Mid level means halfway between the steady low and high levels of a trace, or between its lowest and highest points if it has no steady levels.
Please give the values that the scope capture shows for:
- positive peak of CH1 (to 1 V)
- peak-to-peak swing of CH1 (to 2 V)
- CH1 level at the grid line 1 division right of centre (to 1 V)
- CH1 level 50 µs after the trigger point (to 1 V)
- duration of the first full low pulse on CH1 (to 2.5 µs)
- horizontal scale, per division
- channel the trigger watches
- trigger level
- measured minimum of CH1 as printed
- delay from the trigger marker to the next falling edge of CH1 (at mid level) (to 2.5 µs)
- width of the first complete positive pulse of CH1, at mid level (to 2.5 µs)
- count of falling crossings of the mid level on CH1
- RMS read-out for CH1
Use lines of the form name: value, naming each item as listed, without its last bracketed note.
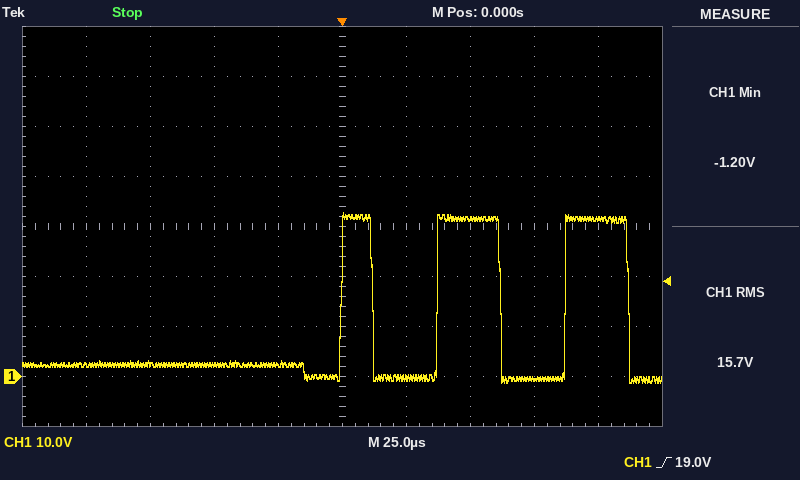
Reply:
positive peak of CH1: 33 V
peak-to-peak swing of CH1: 34 V
CH1 level at the grid line 1 division right of centre: 0 V
CH1 level 50 µs after the trigger point: 32 V
duration of the first full low pulse on CH1: 25.0 µs
horizontal scale, per division: 25 µs
channel the trigger watches: CH1
trigger level: 19.0 V
measured minimum of CH1 as printed: -1.20 V
delay from the trigger marker to the next falling edge of CH1 (at mid level): 12.5 µs
width of the first complete positive pulse of CH1, at mid level: 12.5 µs
count of falling crossings of the mid level on CH1: 3
RMS read-out for CH1: 15.7 V
